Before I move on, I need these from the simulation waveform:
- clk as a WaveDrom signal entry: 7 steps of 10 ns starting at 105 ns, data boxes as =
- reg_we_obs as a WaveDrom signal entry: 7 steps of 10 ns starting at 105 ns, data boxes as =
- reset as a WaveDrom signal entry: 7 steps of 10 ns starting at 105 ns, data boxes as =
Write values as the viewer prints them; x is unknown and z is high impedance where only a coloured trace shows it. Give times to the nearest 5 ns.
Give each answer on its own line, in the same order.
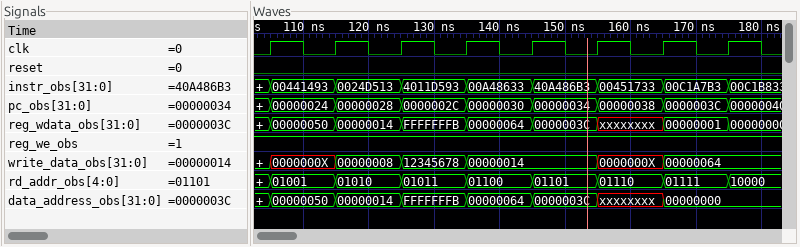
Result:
{name: 'clk', wave: 'p......'}
{name: 'reg_we_obs', wave: '1......'}
{name: 'reset', wave: '0......'}
